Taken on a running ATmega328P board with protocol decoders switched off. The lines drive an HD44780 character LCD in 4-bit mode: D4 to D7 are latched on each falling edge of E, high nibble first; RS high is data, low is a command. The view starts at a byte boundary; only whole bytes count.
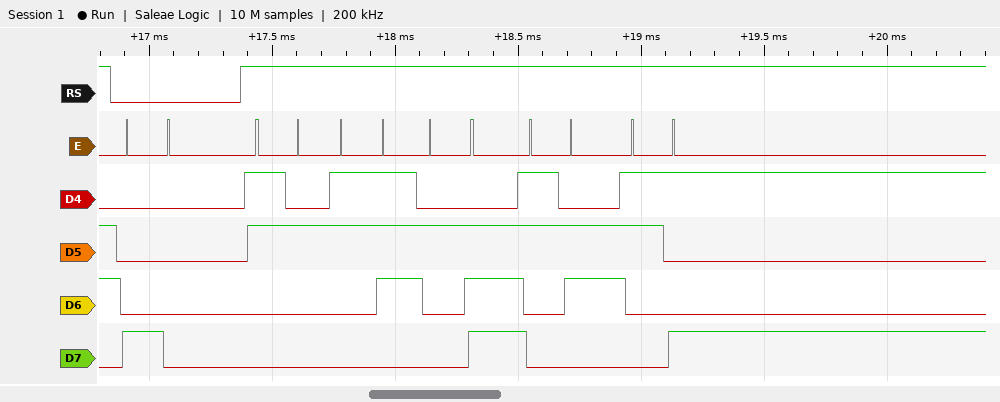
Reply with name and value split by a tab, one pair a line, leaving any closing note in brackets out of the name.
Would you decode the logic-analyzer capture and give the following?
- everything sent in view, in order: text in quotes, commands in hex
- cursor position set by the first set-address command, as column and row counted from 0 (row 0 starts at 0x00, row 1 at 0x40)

everything sent in view, in order: text in quotes, commands in hex	0x80 "27.69"
cursor position set by the first set-address command, as column and row counted from 0	column 0, row 0
